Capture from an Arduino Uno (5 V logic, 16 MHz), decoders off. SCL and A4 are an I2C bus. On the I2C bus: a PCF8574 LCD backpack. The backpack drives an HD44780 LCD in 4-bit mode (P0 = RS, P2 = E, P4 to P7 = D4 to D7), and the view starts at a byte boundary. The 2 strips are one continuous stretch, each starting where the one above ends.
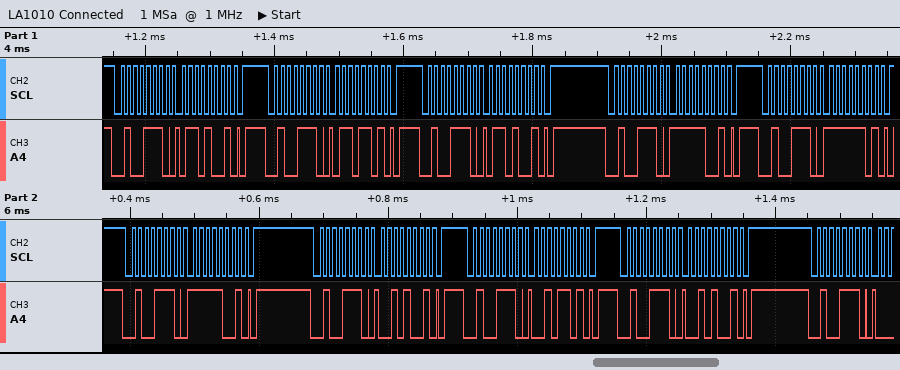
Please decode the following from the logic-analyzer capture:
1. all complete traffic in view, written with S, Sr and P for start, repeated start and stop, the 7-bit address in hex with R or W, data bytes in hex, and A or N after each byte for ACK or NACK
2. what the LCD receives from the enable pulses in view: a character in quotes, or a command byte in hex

S 27W A 69 A P S 27W A 6D A P S 27W A 69 A P S 27W A F9 A P S 27W A FD A P S 27W A F9 A P S 27W A 29 A P S 27W A 2D A P S 27W A 29 A P S 27W A
'o'
